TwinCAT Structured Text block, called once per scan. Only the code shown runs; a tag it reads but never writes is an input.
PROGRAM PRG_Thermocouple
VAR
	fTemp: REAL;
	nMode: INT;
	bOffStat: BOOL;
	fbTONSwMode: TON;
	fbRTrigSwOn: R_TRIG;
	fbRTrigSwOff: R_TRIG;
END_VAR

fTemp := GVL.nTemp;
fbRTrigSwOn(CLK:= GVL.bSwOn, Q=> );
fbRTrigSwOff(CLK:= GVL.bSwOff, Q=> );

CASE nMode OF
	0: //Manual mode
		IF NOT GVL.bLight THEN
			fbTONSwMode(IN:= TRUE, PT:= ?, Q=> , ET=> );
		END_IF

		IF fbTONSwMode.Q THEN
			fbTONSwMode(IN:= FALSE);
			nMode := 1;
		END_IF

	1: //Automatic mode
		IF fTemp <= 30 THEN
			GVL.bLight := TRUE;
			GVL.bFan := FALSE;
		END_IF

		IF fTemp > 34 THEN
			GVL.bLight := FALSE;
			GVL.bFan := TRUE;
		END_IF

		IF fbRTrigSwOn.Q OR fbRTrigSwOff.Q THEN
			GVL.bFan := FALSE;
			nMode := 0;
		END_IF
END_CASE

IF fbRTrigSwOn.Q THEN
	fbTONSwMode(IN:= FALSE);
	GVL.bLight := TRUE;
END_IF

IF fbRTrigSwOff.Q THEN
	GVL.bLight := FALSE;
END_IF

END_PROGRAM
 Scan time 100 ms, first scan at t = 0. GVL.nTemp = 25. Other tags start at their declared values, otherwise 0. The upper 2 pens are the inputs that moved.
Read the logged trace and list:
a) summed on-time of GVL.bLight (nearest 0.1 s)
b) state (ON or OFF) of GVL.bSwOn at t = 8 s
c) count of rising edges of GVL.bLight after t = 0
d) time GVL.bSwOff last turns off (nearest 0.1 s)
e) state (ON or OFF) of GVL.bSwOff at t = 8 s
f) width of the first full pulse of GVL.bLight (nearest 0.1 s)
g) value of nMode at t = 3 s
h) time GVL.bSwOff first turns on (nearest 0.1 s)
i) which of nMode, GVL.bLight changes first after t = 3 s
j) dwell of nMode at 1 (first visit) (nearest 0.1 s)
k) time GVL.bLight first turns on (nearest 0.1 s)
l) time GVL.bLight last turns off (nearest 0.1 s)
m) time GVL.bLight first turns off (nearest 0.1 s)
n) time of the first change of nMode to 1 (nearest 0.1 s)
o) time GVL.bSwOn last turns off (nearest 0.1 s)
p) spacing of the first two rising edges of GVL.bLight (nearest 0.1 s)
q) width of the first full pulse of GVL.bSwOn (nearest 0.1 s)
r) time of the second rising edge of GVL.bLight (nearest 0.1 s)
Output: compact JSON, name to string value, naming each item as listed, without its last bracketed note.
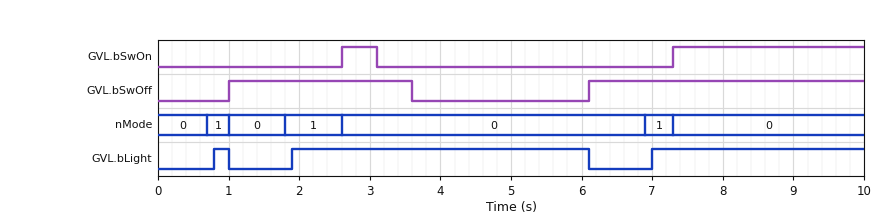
{"summed on-time of GVL.bLight": "7.4 s", "state (ON or OFF) of GVL.bSwOn at t = 8 s": "ON", "count of rising edges of GVL.bLight after t = 0": "3", "time GVL.bSwOff last turns off": "3.6 s", "state (ON or OFF) of GVL.bSwOff at t = 8 s": "ON", "width of the first full pulse of GVL.bLight": "0.2 s", "value of nMode at t = 3 s": "0", "time GVL.bSwOff first turns on": "1.0 s", "which of nMode, GVL.bLight changes first after t = 3 s": "GVL.bLight", "dwell of nMode at 1 (first visit)": "0.3 s", "time GVL.bLight first turns on": "0.8 s", "time GVL.bLight last turns off": "6.1 s", "time GVL.bLight first turns off": "1.0 s", "time of the first change of nMode to 1": "0.7 s", "time GVL.bSwOn last turns off": "3.1 s", "spacing of the first two rising edges of GVL.bLight": "1.1 s", "width of the first full pulse of GVL.bSwOn": "0.5 s", "time of the second rising edge of GVL.bLight": "1.9 s"}
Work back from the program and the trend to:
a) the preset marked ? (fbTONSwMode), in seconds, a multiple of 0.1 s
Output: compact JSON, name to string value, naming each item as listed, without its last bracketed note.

{"the preset marked ? (fbTONSwMode), in seconds, a multiple of 0.1 s": "0.7 s"}
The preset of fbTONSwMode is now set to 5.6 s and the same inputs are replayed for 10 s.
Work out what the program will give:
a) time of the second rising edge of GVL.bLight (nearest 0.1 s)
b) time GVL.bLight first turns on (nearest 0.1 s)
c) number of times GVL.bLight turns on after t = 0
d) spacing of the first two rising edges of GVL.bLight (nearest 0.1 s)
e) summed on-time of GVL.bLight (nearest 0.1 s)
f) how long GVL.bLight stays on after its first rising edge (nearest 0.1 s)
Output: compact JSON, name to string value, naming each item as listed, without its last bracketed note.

{"time of the second rising edge of GVL.bLight": "7.3 s", "time GVL.bLight first turns on": "2.6 s", "number of times GVL.bLight turns on after t = 0": "2", "spacing of the first two rising edges of GVL.bLight": "4.7 s", "summed on-time of GVL.bLight": "6.2 s", "how long GVL.bLight stays on after its first rising edge": "3.5 s"}
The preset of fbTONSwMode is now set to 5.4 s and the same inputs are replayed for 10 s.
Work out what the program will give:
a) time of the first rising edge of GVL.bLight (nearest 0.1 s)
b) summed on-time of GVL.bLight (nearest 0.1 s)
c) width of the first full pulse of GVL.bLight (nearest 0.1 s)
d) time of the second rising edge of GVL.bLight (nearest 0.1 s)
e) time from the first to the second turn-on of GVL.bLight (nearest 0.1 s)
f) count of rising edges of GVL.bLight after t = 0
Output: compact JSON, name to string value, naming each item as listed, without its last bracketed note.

{"time of the first rising edge of GVL.bLight": "2.6 s", "summed on-time of GVL.bLight": "6.2 s", "width of the first full pulse of GVL.bLight": "3.5 s", "time of the second rising edge of GVL.bLight": "7.3 s", "time from the first to the second turn-on of GVL.bLight": "4.7 s", "count of rising edges of GVL.bLight after t = 0": "2"}
